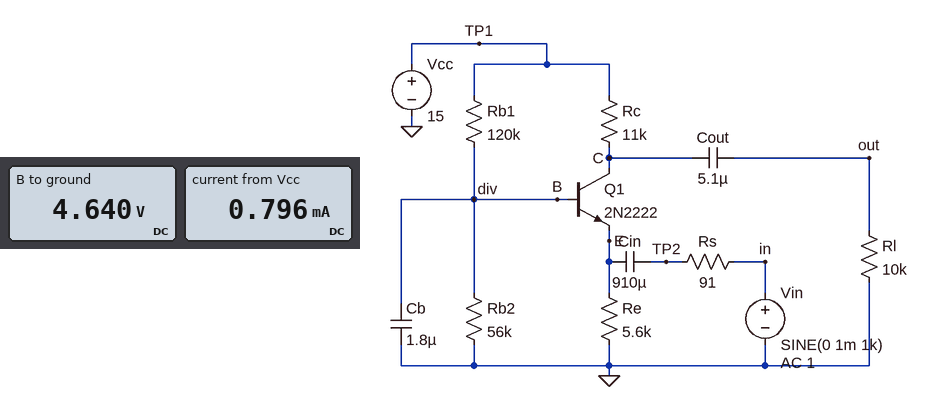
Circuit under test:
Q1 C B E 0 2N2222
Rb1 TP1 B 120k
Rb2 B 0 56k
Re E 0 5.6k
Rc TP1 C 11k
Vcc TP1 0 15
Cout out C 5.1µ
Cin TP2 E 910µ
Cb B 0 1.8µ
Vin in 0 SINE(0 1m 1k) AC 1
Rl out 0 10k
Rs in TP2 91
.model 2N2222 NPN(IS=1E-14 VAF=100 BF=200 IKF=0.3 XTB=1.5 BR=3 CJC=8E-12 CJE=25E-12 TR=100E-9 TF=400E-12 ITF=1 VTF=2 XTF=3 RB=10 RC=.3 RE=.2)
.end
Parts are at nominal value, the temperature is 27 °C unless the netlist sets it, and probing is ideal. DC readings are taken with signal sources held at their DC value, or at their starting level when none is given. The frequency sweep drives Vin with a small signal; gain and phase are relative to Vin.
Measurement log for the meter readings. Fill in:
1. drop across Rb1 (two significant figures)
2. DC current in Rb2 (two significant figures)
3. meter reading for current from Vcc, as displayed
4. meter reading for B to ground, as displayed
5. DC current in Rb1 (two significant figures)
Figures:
10 V
83 µA
0.796 mA
4.640 V
86 µA
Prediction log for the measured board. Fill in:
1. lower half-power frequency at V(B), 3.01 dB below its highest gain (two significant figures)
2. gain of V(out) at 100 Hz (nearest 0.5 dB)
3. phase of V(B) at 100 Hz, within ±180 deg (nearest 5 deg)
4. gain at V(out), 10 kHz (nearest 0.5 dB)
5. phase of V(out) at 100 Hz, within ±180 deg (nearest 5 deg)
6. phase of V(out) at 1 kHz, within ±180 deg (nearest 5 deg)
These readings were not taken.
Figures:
420 mHz
32.0 dB
-85 deg
32.0 dB
5 deg
0 deg
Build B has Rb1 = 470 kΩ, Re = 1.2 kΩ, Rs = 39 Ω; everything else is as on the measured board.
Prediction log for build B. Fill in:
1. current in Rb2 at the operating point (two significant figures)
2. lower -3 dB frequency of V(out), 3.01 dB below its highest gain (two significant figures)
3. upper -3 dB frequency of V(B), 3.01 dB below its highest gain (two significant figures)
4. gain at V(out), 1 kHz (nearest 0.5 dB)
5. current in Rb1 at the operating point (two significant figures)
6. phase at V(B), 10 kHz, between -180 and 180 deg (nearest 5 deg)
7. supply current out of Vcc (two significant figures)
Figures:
26 µA
8.9 Hz
9.9 Hz
36.0 dB
29 µA
-75 deg
690 µA
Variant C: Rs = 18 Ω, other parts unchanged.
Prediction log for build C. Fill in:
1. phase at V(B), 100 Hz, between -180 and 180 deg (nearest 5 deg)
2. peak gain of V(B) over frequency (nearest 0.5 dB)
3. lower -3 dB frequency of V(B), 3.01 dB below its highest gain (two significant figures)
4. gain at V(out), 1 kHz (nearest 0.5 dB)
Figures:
-80 deg
-4.5 dB
520 mHz
39.5 dB
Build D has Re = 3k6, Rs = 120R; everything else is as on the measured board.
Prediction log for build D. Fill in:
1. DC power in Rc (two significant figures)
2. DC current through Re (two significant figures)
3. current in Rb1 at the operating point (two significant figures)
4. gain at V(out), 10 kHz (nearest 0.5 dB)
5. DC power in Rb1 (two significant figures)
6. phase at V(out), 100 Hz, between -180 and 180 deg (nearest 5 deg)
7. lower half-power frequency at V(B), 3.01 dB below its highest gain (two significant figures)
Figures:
11 mW
1.0 mA
89 µA
22.0 dB
940 µW
60 deg
67 mHz
